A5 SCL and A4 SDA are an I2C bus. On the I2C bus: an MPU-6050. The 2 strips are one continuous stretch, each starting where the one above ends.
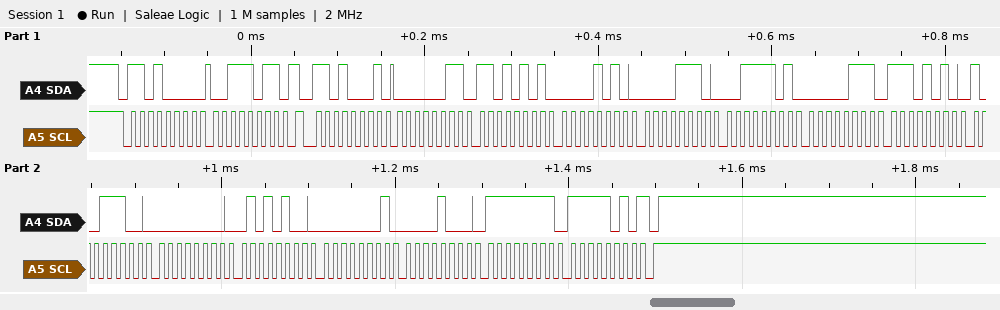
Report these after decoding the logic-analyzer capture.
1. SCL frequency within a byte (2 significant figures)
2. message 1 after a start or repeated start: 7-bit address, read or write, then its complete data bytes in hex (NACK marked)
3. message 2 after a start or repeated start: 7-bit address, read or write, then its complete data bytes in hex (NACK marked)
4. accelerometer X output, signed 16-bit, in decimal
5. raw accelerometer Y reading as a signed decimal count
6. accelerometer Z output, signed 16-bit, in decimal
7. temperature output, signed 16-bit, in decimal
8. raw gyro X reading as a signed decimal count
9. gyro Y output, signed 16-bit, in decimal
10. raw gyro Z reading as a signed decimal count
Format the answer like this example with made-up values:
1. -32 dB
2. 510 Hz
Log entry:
1. 100 kHz
2. 0x68 write: 3B
3. 0x68 read: 03 D5 0A 0E 3D 07 EA 9C 00 54 01 08 FF FA NACK
4. 981
5. 2574
6. 15623
7. -5476
8. 84
9. 264
10. -6
